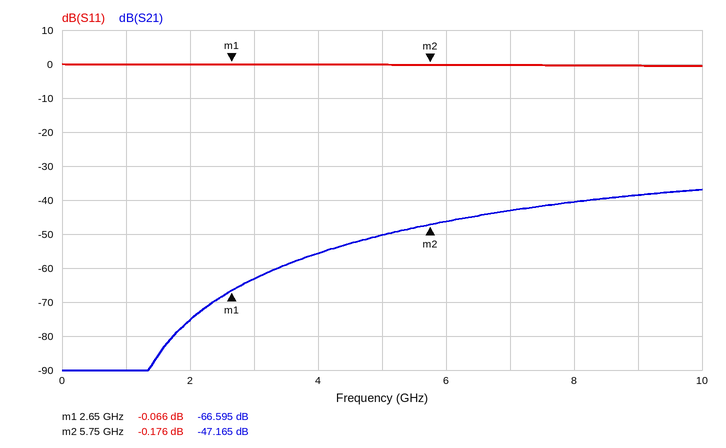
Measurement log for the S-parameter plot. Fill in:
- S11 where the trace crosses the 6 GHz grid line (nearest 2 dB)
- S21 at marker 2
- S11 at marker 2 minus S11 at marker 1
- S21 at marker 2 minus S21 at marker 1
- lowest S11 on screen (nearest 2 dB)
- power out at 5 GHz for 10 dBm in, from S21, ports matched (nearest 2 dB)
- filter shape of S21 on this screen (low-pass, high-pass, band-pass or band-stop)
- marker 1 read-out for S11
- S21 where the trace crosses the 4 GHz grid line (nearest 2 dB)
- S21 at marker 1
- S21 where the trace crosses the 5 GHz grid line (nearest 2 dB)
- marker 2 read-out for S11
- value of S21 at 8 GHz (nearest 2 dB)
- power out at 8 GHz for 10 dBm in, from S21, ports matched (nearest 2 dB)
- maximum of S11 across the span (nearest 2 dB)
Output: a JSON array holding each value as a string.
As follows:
["0 dB", "-47.165 dB", "-0.110 dB", "19.430 dB", "0 dB", "-40 dBm", "high-pass", "-0.066 dB", "-56 dB", "-66.595 dB", "-50 dB", "-0.176 dB", "-40 dB", "-30 dBm", "0 dB"]
